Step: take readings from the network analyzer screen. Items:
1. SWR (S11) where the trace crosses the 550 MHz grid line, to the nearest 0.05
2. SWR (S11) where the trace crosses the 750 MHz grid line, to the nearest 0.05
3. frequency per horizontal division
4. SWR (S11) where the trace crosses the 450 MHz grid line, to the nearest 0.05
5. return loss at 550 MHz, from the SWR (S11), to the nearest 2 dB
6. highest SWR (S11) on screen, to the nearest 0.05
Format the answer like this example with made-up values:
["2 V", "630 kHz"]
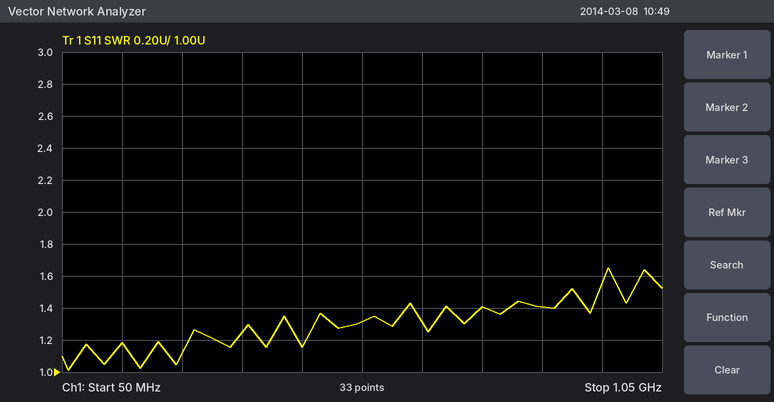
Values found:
["1.30", "1.40", "100 MHz", "1.15", "18 dB", "1.65"]
